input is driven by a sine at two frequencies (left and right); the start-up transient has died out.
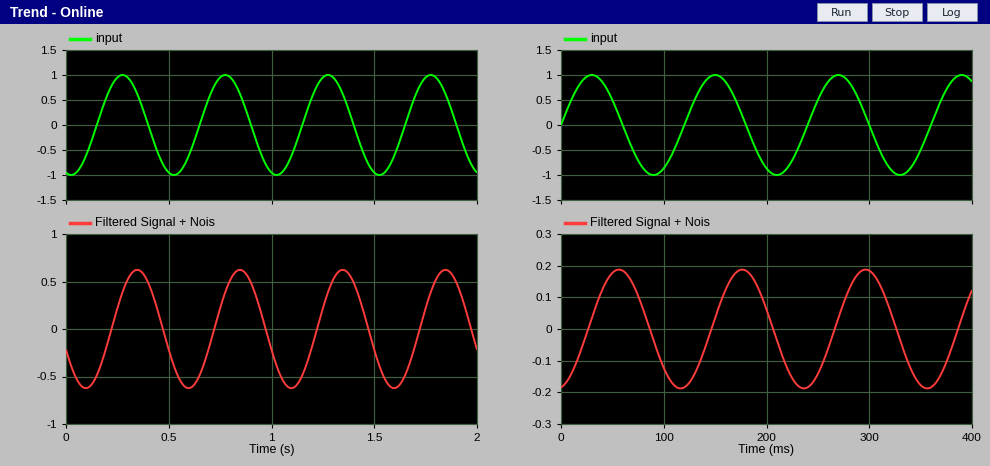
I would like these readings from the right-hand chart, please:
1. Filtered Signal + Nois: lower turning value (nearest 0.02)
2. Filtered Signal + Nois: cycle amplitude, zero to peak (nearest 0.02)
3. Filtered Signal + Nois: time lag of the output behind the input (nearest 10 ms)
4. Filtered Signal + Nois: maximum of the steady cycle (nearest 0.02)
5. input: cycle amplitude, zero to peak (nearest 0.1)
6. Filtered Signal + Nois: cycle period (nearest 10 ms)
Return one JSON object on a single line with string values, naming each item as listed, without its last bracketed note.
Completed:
{"Filtered Signal + Nois: lower turning value": "-0.18", "Filtered Signal + Nois: cycle amplitude, zero to peak": "0.18", "Filtered Signal + Nois: time lag of the output behind the input": "30 ms", "Filtered Signal + Nois: maximum of the steady cycle": "0.18", "input: cycle amplitude, zero to peak": "1.0", "Filtered Signal + Nois: cycle period": "120 ms"}
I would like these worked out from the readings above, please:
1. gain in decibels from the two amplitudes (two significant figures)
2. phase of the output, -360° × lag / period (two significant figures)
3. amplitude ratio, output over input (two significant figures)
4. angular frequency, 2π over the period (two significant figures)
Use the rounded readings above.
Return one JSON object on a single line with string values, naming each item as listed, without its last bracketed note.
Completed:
{"gain in decibels from the two amplitudes": "-15 dB", "phase of the output, -360° × lag / period": "-90°", "amplitude ratio, output over input": "0.18", "angular frequency, 2π over the period": "0.052 rad/ms"}
